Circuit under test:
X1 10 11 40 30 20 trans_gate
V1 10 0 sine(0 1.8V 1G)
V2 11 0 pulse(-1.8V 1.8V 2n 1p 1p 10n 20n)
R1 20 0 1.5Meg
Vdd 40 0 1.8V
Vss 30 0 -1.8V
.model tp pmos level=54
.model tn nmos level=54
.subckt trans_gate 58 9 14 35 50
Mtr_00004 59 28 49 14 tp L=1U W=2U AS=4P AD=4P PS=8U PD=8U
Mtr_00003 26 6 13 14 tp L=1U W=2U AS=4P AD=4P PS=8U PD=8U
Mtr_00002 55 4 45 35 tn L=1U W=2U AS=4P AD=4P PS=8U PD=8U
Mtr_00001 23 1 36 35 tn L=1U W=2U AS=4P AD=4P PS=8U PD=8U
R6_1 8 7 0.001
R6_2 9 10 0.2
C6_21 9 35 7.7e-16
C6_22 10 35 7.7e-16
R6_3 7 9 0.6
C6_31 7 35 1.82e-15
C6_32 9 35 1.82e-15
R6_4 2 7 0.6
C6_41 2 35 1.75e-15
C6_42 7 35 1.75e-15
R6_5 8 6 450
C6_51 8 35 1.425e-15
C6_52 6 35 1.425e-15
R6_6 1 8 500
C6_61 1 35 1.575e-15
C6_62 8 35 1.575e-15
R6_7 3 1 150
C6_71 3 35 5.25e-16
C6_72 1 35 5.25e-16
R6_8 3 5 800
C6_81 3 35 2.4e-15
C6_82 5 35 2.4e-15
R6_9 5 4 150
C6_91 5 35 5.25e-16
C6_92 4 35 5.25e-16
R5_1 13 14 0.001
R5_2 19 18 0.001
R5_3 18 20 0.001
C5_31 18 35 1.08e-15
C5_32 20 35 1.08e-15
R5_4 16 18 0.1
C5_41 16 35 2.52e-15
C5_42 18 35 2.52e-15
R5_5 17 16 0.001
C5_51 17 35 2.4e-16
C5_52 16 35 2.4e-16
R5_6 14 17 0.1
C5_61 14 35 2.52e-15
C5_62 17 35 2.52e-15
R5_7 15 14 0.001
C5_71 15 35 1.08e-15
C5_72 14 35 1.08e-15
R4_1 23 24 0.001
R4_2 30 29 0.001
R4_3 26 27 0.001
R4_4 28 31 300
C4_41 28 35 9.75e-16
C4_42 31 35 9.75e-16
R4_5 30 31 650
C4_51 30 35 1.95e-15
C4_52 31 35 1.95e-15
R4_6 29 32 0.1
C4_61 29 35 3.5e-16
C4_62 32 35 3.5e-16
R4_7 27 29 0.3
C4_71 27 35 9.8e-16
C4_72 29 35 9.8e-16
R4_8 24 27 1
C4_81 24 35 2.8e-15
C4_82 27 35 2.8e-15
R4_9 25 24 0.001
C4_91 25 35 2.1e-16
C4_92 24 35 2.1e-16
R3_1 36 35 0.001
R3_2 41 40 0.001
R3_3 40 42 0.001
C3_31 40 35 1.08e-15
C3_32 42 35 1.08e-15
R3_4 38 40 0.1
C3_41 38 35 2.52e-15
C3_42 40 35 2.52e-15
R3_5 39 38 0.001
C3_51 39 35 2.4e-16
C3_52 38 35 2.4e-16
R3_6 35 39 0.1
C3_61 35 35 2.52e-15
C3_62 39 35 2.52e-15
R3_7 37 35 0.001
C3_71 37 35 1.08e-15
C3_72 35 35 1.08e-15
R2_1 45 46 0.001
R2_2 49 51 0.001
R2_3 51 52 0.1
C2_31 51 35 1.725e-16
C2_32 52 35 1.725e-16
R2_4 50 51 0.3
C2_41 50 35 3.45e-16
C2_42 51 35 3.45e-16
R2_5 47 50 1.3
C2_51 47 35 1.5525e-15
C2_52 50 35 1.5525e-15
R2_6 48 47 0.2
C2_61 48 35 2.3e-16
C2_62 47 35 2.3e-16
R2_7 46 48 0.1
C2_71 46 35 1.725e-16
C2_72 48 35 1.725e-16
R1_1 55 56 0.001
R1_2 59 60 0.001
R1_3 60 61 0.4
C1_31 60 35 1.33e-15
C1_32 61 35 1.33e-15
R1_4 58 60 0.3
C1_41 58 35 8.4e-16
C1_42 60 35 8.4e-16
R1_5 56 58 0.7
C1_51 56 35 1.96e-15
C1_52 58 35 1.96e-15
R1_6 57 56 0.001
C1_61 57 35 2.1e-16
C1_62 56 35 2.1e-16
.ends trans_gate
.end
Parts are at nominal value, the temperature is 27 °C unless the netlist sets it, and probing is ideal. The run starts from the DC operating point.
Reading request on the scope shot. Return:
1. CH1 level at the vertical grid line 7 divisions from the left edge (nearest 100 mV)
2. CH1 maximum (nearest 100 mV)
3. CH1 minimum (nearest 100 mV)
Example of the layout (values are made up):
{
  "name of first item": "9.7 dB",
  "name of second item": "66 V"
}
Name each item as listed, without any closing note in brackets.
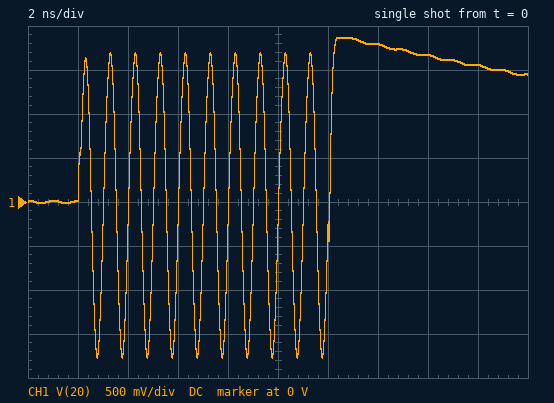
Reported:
{
  "CH1 level at the vertical grid line 7 divisions from the left edge": "1.8 V",
  "CH1 maximum": "1.9 V",
  "CH1 minimum": "-1.8 V"
}
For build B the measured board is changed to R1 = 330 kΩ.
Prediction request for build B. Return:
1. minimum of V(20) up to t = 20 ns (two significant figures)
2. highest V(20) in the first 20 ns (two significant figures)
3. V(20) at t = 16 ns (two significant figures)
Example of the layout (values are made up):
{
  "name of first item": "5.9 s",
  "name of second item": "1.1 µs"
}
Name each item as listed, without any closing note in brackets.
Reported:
{
  "minimum of V(20) up to t = 20 ns": "-1.8 V",
  "highest V(20) in the first 20 ns": "1.8 V",
  "V(20) at t = 16 ns": "1.0 V"
}
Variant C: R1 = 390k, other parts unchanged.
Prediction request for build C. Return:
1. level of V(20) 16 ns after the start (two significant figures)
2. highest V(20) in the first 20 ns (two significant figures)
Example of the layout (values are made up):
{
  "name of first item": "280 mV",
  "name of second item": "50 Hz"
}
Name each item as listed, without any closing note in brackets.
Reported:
{
  "level of V(20) 16 ns after the start": "1.1 V",
  "highest V(20) in the first 20 ns": "1.8 V"
}
